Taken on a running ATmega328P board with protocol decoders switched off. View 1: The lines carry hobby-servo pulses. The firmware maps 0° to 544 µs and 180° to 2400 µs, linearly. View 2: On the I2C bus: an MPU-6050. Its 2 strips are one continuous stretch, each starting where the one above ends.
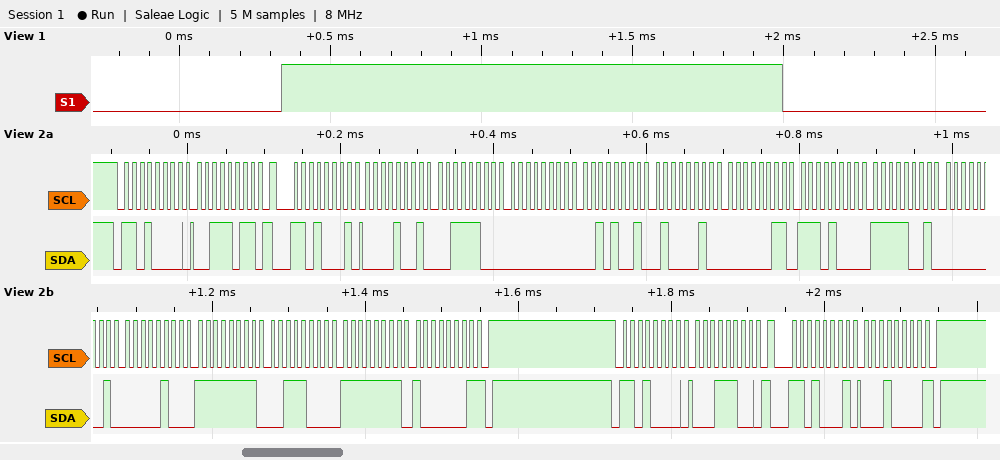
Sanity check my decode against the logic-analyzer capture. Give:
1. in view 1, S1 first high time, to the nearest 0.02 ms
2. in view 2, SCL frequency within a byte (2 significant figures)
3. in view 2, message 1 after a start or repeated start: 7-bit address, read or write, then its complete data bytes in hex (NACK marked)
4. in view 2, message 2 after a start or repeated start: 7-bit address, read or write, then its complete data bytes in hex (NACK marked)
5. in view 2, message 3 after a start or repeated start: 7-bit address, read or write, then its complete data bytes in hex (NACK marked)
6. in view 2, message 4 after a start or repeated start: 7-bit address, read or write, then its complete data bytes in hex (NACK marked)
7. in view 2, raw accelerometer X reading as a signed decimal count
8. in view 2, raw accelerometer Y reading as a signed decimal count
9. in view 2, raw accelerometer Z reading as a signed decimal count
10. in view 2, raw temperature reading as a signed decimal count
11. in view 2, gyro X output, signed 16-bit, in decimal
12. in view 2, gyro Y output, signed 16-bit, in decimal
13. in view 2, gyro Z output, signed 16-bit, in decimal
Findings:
1.66 ms
100 kHz
0x68 write: 3B
0x68 read: 09 3C 00 29 42 03 E8 F9 01 04 FF 38 FF 81 NACK
0x68 write: 1C
0x68 read: 10 NACK
2364
41
16899
-5895
260
-200
-127
